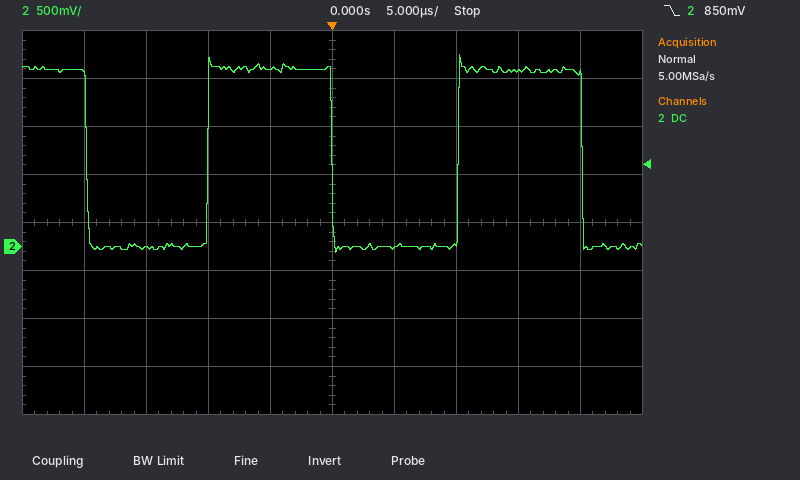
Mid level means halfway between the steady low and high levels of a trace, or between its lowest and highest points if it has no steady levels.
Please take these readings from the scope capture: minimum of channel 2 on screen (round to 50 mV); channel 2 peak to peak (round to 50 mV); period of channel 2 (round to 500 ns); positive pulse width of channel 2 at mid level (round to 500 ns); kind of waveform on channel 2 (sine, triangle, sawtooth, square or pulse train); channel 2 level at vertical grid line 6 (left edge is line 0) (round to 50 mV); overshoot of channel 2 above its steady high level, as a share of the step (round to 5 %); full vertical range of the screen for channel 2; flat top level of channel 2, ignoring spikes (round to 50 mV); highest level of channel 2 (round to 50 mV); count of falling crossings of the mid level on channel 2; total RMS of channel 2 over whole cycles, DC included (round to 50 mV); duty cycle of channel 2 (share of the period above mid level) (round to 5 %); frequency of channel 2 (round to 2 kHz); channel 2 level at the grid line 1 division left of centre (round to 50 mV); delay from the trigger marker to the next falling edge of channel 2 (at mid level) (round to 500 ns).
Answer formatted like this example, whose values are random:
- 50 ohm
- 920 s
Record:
- -50 mV
- 2.05 V
- 20.0 µs
- 10.0 µs
- square
- 0 mV
- 10 %
- 4 V
- 1.85 V
- 2.00 V
- 3
- 1.30 V
- 50 %
- 50 kHz
- 1.85 V
- 20.0 µs
